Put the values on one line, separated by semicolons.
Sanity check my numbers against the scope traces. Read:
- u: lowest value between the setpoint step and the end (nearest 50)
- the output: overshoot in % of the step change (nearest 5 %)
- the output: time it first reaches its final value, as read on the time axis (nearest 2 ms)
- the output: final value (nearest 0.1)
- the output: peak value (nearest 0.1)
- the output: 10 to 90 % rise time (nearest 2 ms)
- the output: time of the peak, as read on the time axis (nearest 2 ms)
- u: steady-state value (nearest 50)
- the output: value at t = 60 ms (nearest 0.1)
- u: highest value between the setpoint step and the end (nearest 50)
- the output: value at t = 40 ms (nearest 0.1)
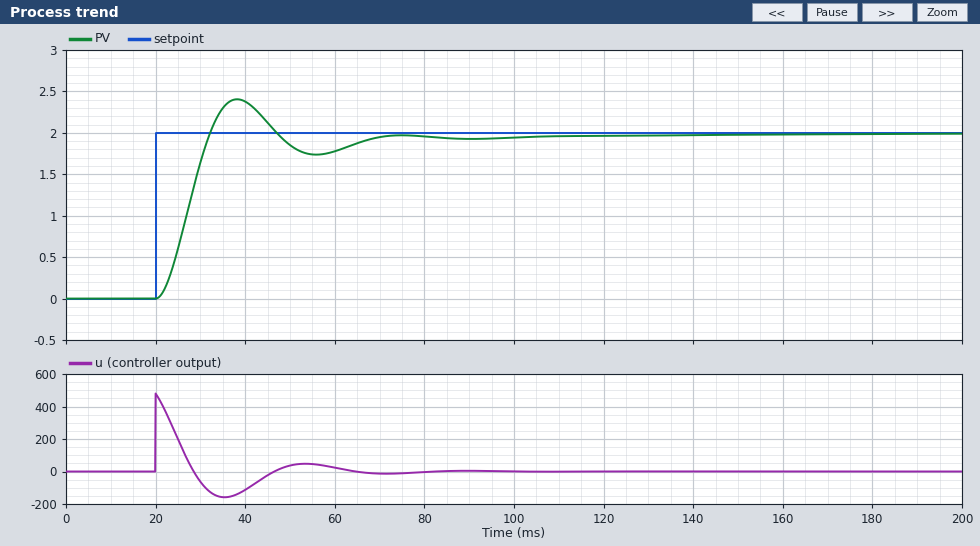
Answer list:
-150; 20 %; 32 ms; 2.0; 2.4; 8 ms; 38 ms; 0; 1.8; 500; 2.4
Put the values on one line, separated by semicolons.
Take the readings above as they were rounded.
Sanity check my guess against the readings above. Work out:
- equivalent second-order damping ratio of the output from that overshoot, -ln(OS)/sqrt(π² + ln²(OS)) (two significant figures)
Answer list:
0.46
